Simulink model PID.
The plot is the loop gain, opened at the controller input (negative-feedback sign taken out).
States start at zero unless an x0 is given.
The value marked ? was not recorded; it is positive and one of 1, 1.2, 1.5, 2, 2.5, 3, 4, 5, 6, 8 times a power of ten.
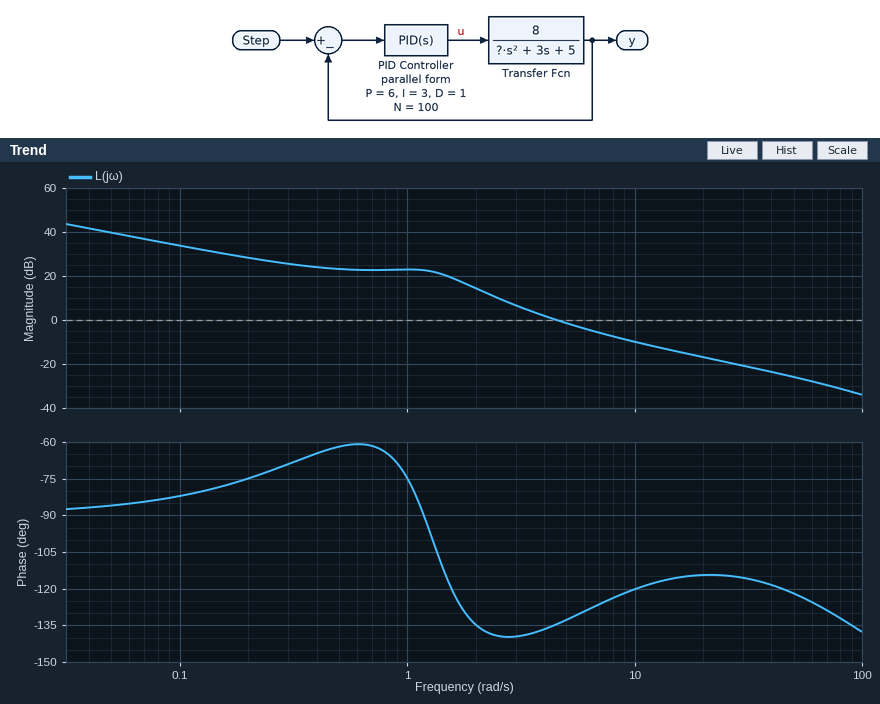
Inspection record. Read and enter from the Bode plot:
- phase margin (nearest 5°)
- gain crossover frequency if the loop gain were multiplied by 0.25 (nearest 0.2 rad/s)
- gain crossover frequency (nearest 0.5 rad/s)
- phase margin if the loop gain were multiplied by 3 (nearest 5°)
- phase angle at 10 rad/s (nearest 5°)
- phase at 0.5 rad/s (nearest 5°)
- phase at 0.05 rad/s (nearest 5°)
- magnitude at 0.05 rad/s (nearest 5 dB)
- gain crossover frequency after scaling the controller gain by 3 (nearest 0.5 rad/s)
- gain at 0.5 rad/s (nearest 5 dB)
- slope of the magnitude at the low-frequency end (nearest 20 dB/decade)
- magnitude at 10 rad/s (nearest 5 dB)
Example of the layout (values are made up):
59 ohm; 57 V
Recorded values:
45°; 2.2 rad/s; 4.5 rad/s; 60°; -120°; -60°; -85°; 40 dB; 9.5 rad/s; 25 dB; -20 dB/decade; -10 dB
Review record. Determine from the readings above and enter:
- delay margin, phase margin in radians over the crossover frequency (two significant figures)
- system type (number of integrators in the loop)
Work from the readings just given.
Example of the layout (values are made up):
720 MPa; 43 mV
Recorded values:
0.17 s; 1
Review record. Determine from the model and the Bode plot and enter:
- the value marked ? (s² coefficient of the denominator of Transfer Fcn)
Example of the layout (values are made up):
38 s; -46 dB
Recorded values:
3
